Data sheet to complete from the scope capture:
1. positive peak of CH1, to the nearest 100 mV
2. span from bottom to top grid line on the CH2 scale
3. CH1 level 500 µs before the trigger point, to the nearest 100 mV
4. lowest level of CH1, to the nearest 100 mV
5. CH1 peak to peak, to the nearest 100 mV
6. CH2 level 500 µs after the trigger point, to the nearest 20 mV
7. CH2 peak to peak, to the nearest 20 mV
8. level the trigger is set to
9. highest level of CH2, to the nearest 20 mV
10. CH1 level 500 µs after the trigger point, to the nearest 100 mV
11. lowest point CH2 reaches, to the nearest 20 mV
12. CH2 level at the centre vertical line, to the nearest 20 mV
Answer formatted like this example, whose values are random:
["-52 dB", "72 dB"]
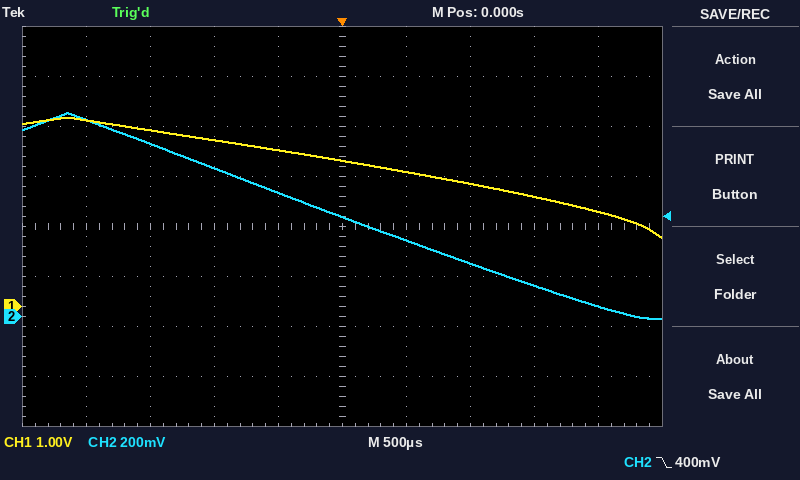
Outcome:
["3.8 V", "1.6 V", "3.1 V", "1.4 V", "2.4 V", "300 mV", "820 mV", "400 mV", "820 mV", "2.7 V", "0 mV", "400 mV"]
